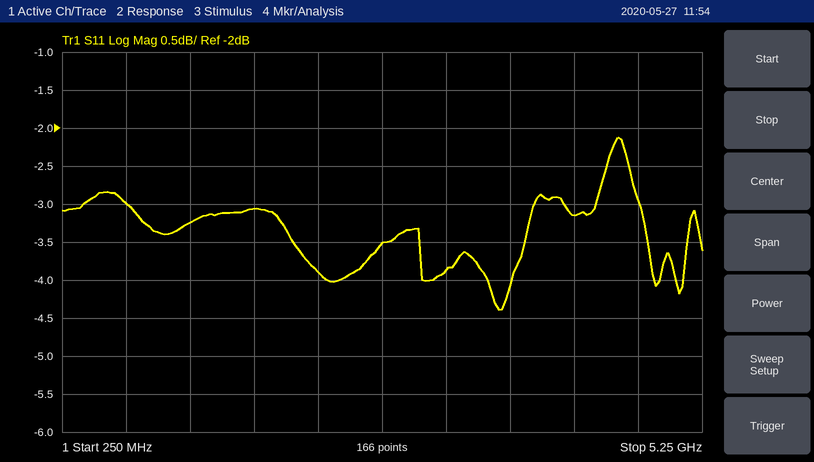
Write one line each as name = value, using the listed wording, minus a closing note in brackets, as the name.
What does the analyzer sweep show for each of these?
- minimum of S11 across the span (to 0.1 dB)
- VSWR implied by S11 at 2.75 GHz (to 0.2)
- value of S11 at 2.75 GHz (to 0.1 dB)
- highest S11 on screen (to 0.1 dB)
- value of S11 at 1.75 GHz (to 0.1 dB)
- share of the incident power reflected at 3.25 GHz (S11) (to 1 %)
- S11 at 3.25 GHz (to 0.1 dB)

minimum of S11 across the span = -4.4 dB
VSWR implied by S11 at 2.75 GHz = 5.0
value of S11 at 2.75 GHz = -3.5 dB
highest S11 on screen = -2.1 dB
value of S11 at 1.75 GHz = -3.1 dB
share of the incident power reflected at 3.25 GHz (S11) = 41 %
S11 at 3.25 GHz = -3.9 dB
